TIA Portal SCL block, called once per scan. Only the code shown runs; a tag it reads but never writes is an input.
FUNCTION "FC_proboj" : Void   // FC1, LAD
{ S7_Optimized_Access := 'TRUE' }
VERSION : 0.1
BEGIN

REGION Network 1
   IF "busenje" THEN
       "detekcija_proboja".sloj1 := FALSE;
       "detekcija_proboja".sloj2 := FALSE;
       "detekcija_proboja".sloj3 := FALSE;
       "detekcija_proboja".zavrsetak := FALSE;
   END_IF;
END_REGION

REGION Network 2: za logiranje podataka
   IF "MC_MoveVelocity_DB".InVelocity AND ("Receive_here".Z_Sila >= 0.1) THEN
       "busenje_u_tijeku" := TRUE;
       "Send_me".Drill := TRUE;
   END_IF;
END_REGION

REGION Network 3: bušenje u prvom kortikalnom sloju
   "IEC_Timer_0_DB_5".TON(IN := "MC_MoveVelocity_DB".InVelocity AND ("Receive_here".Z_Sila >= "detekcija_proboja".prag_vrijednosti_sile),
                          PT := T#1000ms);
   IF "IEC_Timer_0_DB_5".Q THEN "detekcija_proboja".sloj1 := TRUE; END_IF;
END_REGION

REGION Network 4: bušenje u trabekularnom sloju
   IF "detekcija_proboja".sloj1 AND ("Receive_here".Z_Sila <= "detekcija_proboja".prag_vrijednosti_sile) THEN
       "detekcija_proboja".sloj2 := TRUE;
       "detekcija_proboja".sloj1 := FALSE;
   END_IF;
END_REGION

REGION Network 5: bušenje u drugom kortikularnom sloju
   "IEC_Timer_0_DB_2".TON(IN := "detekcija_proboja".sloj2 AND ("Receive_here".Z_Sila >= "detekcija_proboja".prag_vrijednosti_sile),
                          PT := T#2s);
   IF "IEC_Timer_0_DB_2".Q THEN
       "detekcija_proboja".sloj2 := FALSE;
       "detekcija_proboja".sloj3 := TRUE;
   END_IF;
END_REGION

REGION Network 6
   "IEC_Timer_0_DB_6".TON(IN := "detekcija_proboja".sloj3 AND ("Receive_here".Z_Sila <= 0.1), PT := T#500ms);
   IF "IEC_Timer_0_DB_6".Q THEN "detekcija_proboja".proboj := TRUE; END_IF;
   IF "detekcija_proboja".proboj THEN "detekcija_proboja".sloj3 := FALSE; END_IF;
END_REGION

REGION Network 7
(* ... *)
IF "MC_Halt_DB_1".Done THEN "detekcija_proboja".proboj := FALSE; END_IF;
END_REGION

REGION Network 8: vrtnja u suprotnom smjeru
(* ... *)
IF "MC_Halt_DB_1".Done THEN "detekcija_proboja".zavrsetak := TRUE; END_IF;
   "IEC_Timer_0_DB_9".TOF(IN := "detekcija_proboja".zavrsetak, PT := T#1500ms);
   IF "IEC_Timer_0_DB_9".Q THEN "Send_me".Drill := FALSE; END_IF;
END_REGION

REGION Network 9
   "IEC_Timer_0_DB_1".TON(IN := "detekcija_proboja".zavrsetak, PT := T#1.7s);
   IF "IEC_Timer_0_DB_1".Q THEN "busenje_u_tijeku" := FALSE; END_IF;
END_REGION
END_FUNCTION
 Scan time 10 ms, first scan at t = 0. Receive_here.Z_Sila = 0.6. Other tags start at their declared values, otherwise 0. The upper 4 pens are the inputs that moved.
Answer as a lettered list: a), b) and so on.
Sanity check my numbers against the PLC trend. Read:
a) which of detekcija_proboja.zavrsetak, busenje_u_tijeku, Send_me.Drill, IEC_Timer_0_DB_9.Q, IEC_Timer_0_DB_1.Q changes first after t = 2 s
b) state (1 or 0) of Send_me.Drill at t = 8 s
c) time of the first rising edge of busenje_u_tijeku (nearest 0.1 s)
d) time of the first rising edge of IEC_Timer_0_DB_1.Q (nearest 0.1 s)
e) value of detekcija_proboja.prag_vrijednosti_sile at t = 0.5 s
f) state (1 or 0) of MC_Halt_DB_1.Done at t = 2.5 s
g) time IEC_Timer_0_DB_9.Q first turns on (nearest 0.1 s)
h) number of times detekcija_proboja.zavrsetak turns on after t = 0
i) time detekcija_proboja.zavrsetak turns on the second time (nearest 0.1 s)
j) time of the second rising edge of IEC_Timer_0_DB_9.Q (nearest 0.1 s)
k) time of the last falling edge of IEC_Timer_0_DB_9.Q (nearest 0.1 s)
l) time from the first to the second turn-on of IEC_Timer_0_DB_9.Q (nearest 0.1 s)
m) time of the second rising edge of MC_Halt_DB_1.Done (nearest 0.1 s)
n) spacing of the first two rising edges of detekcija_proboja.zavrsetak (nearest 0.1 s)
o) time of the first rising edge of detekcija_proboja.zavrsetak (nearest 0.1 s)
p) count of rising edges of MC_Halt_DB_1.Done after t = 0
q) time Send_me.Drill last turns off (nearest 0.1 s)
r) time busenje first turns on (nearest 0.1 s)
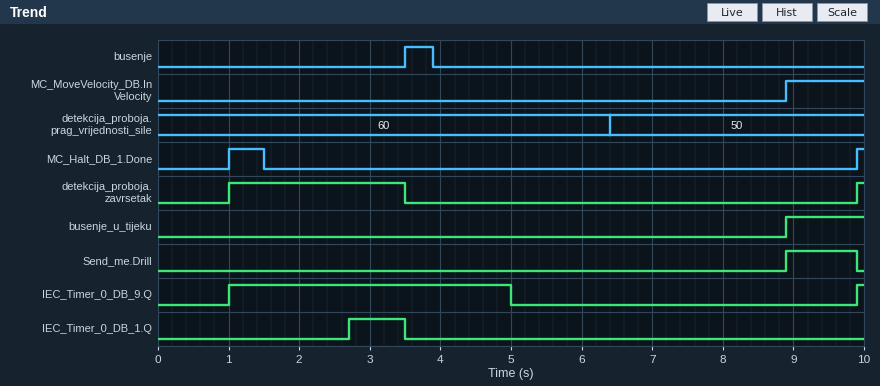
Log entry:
a) IEC_Timer_0_DB_1.Q
b) 0
c) 8.9 s
d) 2.7 s
e) 60
f) 0
g) 1.0 s
h) 2
i) 9.9 s
j) 9.9 s
k) 5.0 s
l) 8.9 s
m) 9.9 s
n) 8.9 s
o) 1.0 s
p) 2
q) 9.9 s
r) 3.5 s
